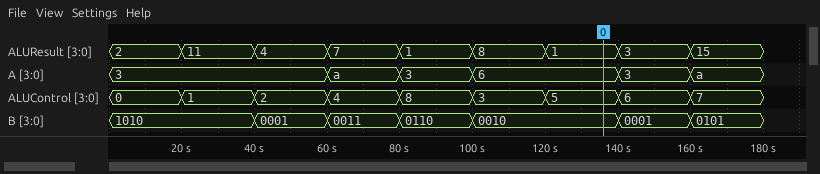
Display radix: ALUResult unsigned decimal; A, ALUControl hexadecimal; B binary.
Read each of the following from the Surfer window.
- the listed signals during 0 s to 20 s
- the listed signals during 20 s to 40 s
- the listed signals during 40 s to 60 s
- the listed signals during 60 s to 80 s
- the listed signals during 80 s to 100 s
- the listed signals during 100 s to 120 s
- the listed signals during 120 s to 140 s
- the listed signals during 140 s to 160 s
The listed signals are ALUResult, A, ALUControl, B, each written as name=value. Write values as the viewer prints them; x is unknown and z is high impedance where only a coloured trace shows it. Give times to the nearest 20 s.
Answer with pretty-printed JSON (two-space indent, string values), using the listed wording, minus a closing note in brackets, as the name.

{
  "the listed signals during 0 s to 20 s": "ALUResult=2, A=3, ALUControl=0, B=1010",
  "the listed signals during 20 s to 40 s": "ALUResult=11, A=3, ALUControl=1, B=1010",
  "the listed signals during 40 s to 60 s": "ALUResult=4, A=3, ALUControl=2, B=0001",
  "the listed signals during 60 s to 80 s": "ALUResult=7, A=a, ALUControl=4, B=0011",
  "the listed signals during 80 s to 100 s": "ALUResult=1, A=3, ALUControl=8, B=0110",
  "the listed signals during 100 s to 120 s": "ALUResult=8, A=6, ALUControl=3, B=0010",
  "the listed signals during 120 s to 140 s": "ALUResult=1, A=6, ALUControl=5, B=0010",
  "the listed signals during 140 s to 160 s": "ALUResult=3, A=3, ALUControl=6, B=0001"
}
